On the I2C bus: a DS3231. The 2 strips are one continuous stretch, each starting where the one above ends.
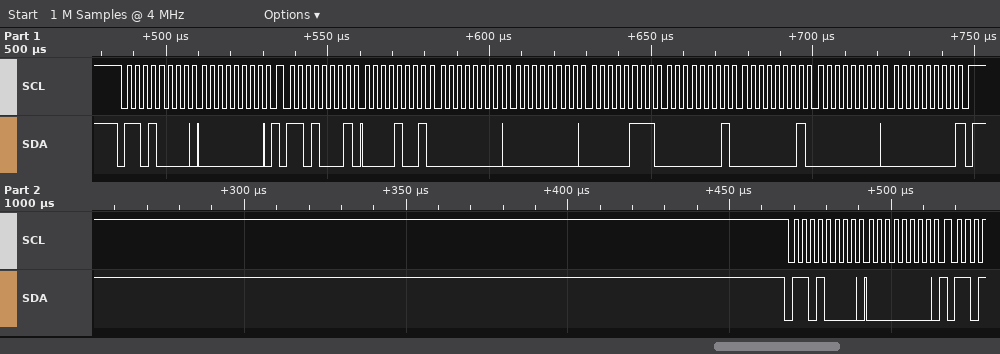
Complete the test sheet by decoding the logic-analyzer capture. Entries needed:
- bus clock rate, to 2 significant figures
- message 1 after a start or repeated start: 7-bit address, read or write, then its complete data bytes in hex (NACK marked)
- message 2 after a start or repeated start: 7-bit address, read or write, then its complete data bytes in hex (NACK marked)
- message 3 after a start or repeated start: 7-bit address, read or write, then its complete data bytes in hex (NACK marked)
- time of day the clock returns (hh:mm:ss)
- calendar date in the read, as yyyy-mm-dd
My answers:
400 kHz
0x68 write: 00
0x68 read: 09 00 00 07 01 01 00 00 NACK
0x68 write: 00
00:00:09
2000-01-01
